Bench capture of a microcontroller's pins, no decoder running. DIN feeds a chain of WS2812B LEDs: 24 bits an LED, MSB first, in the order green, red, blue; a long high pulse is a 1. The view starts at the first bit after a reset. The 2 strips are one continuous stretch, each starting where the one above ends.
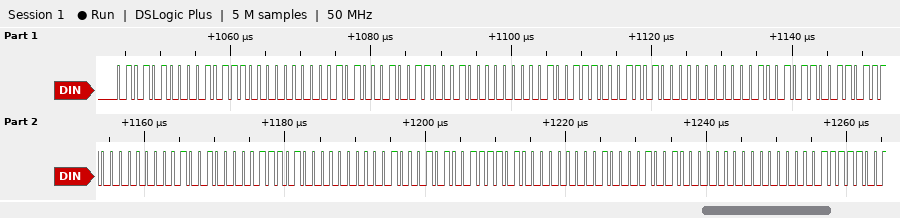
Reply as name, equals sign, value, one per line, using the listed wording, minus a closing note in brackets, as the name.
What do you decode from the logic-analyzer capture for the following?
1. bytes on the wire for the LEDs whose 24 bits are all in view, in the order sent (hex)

bytes on the wire for the LEDs whose 24 bits are all in view, in the order sent = 54 2E 00 51 31 00 4E 34 00 4B 37 00 48 3A 00 45 3D 00 42 40 00
